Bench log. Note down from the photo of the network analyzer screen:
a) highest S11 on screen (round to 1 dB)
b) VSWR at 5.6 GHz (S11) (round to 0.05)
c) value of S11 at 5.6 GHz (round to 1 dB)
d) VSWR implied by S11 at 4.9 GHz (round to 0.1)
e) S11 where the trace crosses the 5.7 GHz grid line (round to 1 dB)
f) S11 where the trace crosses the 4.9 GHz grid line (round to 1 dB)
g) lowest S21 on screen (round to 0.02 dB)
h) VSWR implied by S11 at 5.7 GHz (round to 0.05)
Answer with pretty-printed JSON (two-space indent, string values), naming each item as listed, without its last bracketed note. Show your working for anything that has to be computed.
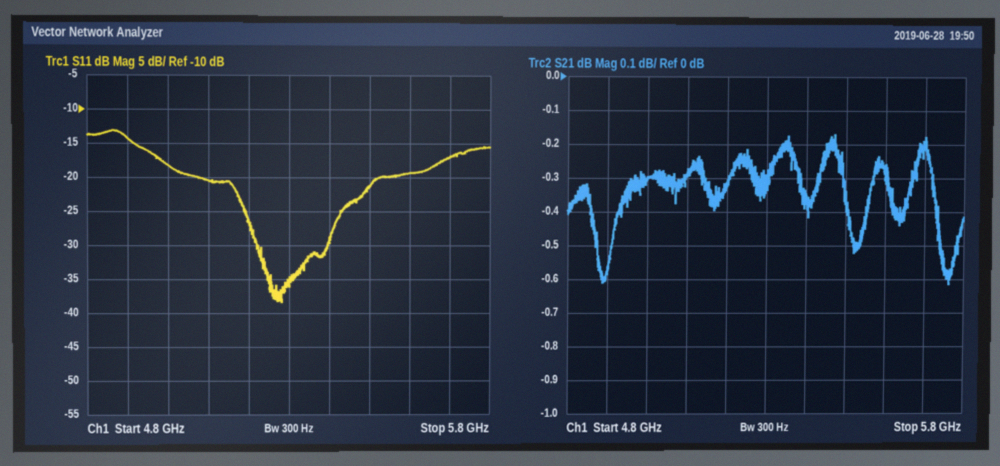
{
  "highest S11 on screen": "-13 dB",
  "VSWR at 5.6 GHz (S11)": "|Γ| = 10^(-19/20) = 0.1122; VSWR = (1 + 0.1122)/(1 − 0.1122) ≈ 1.25",
  "value of S11 at 5.6 GHz": "-19 dB",
  "VSWR implied by S11 at 4.9 GHz": "|Γ| = 10^(-14/20) = 0.1995; VSWR = (1 + 0.1995)/(1 − 0.1995) ≈ 1.5",
  "S11 where the trace crosses the 5.7 GHz grid line": "-17 dB",
  "S11 where the trace crosses the 4.9 GHz grid line": "-14 dB",
  "lowest S21 on screen": "-0.62 dB",
  "VSWR implied by S11 at 5.7 GHz": "|Γ| = 10^(-17/20) = 0.1413; VSWR = (1 + 0.1413)/(1 − 0.1413) ≈ 1.33, so 1.35 to the nearest 0.05"
}
